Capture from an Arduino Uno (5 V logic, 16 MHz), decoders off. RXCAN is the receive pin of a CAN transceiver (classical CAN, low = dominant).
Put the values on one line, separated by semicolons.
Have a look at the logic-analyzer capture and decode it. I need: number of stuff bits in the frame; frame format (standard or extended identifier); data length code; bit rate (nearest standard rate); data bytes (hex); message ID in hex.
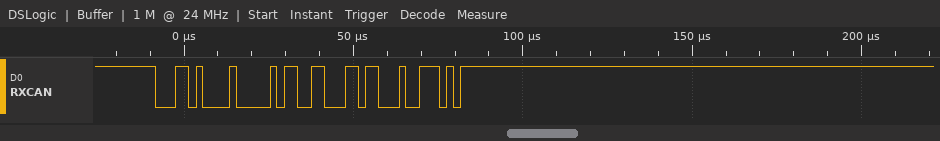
1; standard; 1; 500 kbit/s; 98; 0x1A1
